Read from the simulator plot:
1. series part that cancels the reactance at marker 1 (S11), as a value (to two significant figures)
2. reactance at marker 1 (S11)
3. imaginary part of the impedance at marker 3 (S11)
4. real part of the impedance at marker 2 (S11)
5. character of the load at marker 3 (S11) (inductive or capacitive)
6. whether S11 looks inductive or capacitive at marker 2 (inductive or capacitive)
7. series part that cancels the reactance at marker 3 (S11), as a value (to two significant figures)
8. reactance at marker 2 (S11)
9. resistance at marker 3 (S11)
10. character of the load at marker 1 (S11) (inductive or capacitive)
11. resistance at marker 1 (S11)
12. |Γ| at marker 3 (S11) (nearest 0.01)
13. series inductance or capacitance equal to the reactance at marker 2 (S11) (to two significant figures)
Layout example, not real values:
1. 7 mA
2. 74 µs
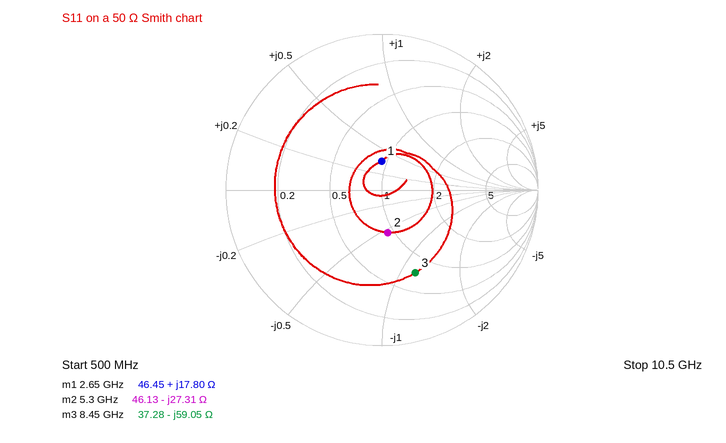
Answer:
1. 3.4 pF
2. +17.80 Ω
3. -59.05 Ω
4. 46.13 Ω
5. capacitive
6. capacitive
7. 1.1 nH
8. -27.31 Ω
9. 37.28 Ω
10. inductive
11. 46.45 Ω
12. 0.57
13. 1.1 pF
